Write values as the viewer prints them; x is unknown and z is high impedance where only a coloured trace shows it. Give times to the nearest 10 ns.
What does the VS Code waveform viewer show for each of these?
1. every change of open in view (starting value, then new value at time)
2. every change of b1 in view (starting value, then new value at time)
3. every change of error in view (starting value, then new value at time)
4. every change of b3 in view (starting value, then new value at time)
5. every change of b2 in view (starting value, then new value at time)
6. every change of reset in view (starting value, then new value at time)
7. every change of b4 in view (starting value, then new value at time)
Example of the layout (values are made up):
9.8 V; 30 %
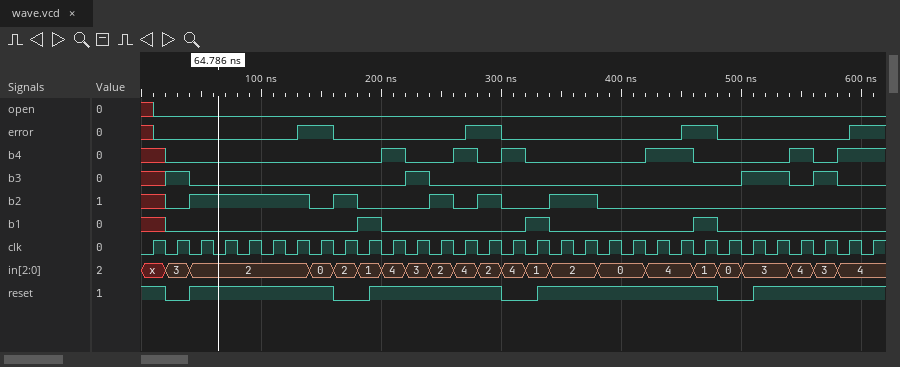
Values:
x, 0 at 10 ns; x, 0 at 20 ns, 1 at 180 ns, 0 at 200 ns, 1 at 320 ns, 0 at 340 ns, 1 at 460 ns, 0 at 480 ns; x, 0 at 10 ns, 1 at 130 ns, 0 at 160 ns, 1 at 270 ns, 0 at 300 ns, 1 at 450 ns, 0 at 480 ns, 1 at 590 ns; x, 1 at 20 ns, 0 at 40 ns, 1 at 220 ns, 0 at 240 ns, 1 at 500 ns, 0 at 540 ns, 1 at 560 ns, 0 at 580 ns; x, 0 at 20 ns, 1 at 40 ns, 0 at 140 ns, 1 at 160 ns, 0 at 180 ns, 1 at 240 ns, 0 at 260 ns, 1 at 280 ns, 0 at 300 ns, 1 at 340 ns, 0 at 380 ns; 1, 0 at 20 ns, 1 at 40 ns, 0 at 160 ns, 1 at 190 ns, 0 at 300 ns, 1 at 330 ns, 0 at 480 ns, 1 at 510 ns; x, 0 at 20 ns, 1 at 200 ns, 0 at 220 ns, 1 at 260 ns, 0 at 280 ns, 1 at 300 ns, 0 at 320 ns, 1 at 420 ns, 0 at 460 ns, 1 at 540 ns, 0 at 560 ns, 1 at 580 ns
